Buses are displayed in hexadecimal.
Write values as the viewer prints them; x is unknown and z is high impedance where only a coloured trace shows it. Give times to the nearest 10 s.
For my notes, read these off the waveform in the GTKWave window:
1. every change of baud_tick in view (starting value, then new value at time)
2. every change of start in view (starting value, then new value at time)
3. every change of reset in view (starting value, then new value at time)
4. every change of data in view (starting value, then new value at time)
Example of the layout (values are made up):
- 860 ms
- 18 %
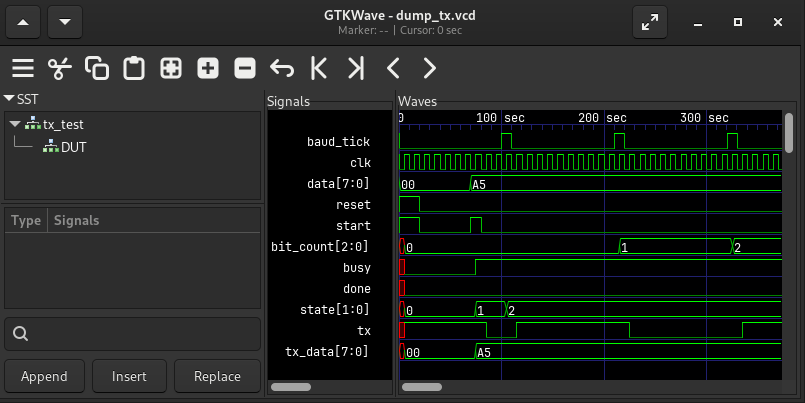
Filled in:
- 0, 1 at 100 s, 0 at 110 s, 1 at 210 s, 0 at 220 s, 1 at 320 s, 0 at 330 s
- 1, 0 at 20 s, 1 at 70 s, 0 at 80 s
- 1, 0 at 20 s
- 00, A5 at 70 s
